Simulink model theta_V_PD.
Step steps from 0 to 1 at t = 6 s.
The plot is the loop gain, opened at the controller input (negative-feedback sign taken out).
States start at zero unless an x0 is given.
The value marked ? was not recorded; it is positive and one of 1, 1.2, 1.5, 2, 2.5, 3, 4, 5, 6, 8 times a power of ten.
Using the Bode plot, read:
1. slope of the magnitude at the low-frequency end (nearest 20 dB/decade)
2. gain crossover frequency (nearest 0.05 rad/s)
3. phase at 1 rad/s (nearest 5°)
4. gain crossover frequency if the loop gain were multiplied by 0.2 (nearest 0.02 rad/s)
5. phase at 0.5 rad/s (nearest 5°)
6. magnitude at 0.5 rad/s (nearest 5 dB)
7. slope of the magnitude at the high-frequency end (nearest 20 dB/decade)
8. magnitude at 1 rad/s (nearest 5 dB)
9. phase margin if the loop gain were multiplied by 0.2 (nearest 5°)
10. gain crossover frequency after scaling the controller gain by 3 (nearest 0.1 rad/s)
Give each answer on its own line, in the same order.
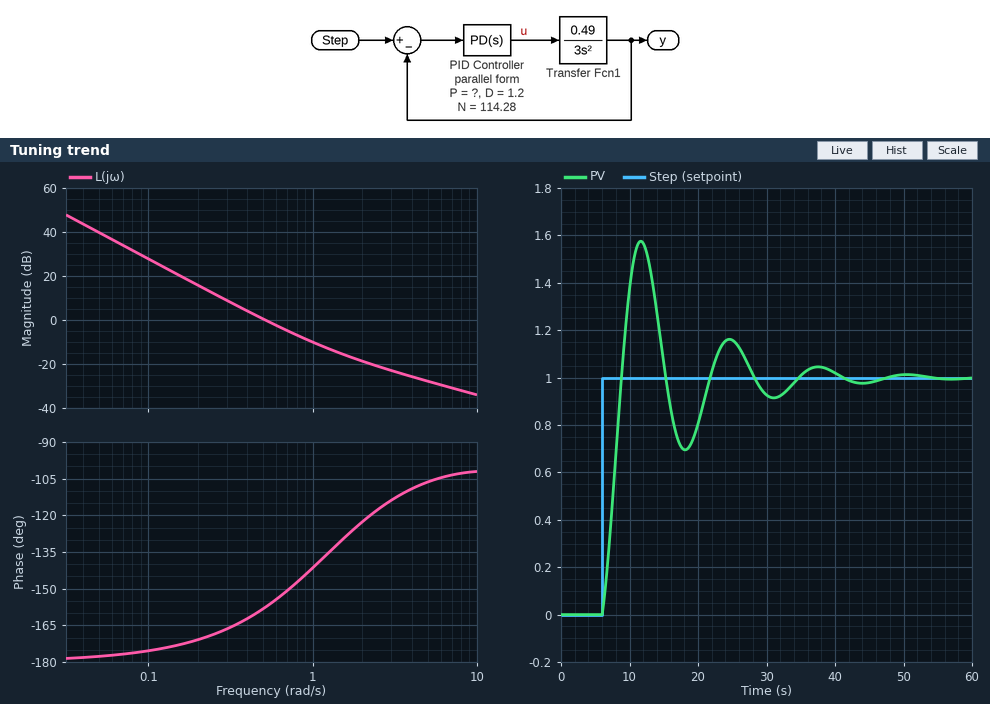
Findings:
-40 dB/decade
0.50 rad/s
-140°
0.22 rad/s
-160°
0 dB
-20 dB/decade
-10 dB
10°
1.0 rad/s
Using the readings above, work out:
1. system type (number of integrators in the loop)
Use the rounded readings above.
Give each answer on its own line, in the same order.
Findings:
2
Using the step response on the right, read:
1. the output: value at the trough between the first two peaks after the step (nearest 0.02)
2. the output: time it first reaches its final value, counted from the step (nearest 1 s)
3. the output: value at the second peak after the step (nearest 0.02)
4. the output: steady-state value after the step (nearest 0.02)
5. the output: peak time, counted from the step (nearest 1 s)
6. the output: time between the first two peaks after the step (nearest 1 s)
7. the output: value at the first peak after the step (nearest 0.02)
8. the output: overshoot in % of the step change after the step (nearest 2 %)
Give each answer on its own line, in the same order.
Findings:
0.70
3 s
1.16
1.00
6 s
13 s
1.58
58 %
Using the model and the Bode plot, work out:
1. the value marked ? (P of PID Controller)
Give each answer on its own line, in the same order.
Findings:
1.5
